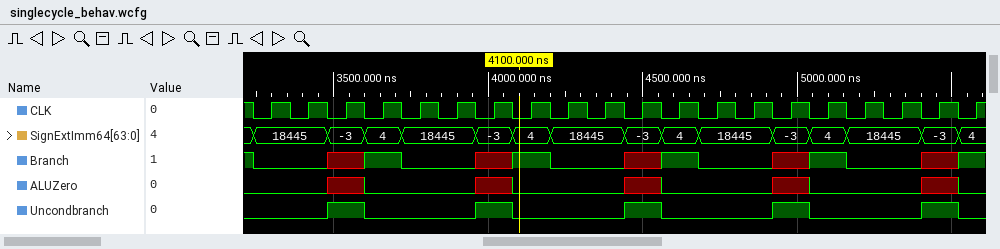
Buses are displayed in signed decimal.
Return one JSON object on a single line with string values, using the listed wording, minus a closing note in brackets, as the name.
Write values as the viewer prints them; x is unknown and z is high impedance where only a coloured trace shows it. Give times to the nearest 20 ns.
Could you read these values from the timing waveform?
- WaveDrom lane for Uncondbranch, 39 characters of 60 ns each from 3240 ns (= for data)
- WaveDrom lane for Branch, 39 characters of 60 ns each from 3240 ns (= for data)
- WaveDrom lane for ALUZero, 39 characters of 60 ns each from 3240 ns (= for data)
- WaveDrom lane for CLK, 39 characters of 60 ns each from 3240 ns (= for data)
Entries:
{"WaveDrom lane for Uncondbranch, 39 characters of 60 ns each from 3240 ns": "{name: 'Uncondbranch', wave: '0...1.0.....1.0.....1.0.....1.0.....1.0'}", "WaveDrom lane for Branch, 39 characters of 60 ns each from 3240 ns": "{name: 'Branch', wave: '0...x.1.0...x.1.0...x.1.0...x.1.0...x.1'}", "WaveDrom lane for ALUZero, 39 characters of 60 ns each from 3240 ns": "{name: 'ALUZero', wave: '0...x.0.....x.0.....x.0.....x.0.....x.0'}", "WaveDrom lane for CLK, 39 characters of 60 ns each from 3240 ns": "{name: 'CLK', wave: '010101010101010101010101010101010101010'}"}
